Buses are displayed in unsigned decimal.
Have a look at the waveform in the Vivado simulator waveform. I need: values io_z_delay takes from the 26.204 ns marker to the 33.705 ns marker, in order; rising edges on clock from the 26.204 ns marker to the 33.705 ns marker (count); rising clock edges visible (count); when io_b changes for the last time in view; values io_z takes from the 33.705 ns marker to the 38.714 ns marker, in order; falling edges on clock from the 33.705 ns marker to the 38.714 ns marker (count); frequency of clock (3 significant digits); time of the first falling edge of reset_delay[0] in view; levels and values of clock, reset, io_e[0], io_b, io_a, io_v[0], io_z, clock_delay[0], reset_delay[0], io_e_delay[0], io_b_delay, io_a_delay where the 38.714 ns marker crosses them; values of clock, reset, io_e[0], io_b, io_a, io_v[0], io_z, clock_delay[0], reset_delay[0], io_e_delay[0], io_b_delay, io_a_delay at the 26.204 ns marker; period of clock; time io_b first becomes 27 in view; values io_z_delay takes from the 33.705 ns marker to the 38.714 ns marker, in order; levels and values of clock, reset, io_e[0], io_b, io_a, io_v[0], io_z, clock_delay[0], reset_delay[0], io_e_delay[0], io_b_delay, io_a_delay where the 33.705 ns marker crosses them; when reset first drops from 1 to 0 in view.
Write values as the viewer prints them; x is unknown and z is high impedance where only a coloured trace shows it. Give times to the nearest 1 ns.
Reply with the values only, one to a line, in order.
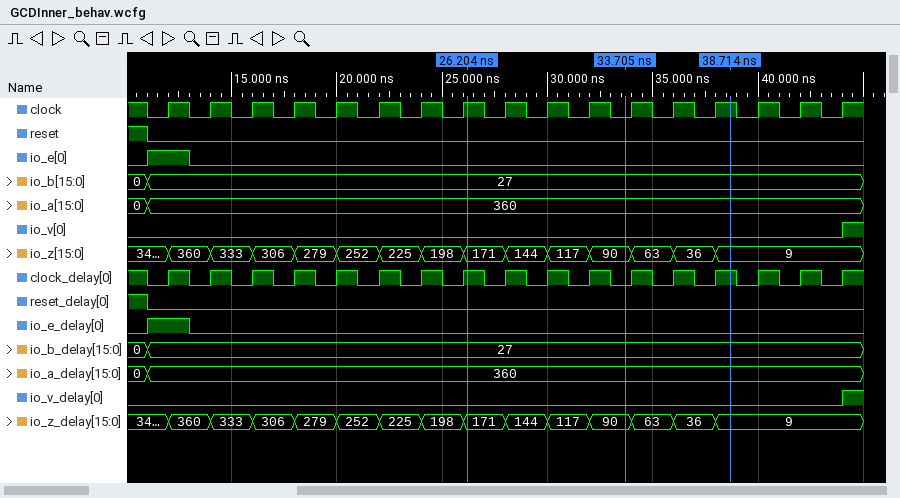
171, 144, 117, 90
3
17
11 ns
90, 63, 36, 9
2
500 MHz
11 ns
clock=1, reset=0, io_e[0]=0, io_b=27, io_a=360, io_v[0]=0, io_z=9, clock_delay[0]=1, reset_delay[0]=0, io_e_delay[0]=0, io_b_delay=27, io_a_delay=360
clock=1, reset=0, io_e[0]=0, io_b=27, io_a=360, io_v[0]=0, io_z=171, clock_delay[0]=1, reset_delay[0]=0, io_e_delay[0]=0, io_b_delay=27, io_a_delay=360
2 ns
11 ns
90, 63, 36, 9
clock=0, reset=0, io_e[0]=0, io_b=27, io_a=360, io_v[0]=0, io_z=90, clock_delay[0]=0, reset_delay[0]=0, io_e_delay[0]=0, io_b_delay=27, io_a_delay=360
11 ns
